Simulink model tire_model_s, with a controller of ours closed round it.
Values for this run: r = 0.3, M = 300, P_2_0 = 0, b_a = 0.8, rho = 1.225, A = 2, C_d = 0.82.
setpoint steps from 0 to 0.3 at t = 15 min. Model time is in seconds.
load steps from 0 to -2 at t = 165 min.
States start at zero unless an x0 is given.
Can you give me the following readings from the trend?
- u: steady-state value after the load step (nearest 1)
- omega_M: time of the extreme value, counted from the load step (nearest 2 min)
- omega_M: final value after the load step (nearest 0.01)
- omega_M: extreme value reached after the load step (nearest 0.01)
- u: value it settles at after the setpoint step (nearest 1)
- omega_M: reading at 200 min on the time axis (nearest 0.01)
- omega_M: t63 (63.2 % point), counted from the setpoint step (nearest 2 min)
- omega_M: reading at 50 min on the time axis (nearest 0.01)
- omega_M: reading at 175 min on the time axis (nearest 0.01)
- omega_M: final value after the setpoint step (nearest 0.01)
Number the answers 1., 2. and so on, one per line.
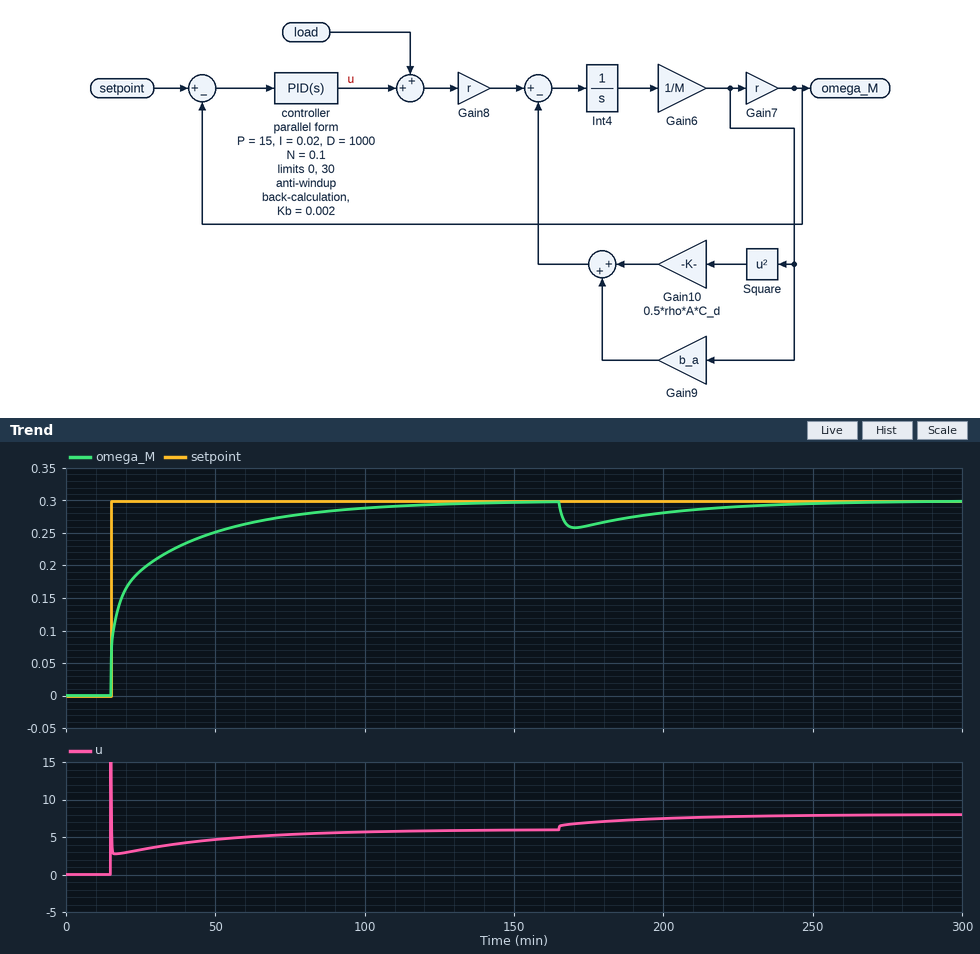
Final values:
1. 8
2. 6 min
3. 0.30
4. 0.26
5. 6
6. 0.28
7. 10 min
8. 0.25
9. 0.26
10. 0.30
